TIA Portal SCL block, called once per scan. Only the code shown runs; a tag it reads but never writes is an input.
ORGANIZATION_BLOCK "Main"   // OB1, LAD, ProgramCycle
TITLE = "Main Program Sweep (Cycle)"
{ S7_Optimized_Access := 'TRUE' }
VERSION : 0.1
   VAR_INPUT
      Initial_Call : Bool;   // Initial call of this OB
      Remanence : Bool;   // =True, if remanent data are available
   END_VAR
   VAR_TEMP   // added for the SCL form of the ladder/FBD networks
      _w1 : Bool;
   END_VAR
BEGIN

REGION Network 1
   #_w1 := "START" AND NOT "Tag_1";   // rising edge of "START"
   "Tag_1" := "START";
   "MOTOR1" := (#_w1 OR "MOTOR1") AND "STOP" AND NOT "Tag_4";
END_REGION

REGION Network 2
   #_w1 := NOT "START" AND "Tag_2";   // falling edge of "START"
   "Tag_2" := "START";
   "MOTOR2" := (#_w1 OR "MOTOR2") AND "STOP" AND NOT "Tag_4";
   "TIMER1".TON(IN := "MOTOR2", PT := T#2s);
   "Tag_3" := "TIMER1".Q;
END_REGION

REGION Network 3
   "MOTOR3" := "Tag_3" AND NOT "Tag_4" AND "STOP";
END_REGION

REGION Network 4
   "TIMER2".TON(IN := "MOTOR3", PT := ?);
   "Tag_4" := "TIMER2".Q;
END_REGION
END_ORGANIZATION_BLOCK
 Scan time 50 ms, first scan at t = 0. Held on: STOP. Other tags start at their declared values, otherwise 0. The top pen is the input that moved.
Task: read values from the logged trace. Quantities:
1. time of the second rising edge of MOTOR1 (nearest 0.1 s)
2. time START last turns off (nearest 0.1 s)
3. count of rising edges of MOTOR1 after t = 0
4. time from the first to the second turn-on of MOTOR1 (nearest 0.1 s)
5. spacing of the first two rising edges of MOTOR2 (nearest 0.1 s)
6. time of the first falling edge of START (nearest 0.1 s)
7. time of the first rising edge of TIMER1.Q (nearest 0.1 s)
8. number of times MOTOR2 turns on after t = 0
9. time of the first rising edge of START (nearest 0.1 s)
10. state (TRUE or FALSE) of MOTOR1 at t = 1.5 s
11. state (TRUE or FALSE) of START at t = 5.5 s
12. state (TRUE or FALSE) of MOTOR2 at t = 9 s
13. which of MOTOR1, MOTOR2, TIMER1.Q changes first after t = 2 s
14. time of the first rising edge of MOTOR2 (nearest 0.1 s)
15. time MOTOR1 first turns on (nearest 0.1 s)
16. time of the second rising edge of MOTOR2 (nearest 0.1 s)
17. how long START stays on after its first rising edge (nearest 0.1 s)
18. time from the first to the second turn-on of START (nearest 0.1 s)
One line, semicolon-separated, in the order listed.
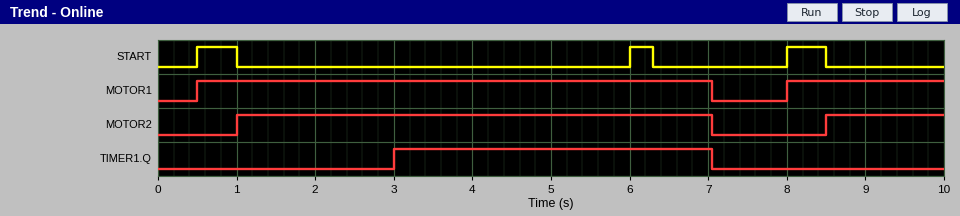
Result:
8.0 s; 8.5 s; 2; 7.5 s; 7.5 s; 1.0 s; 3.0 s; 2; 0.5 s; TRUE; FALSE; TRUE; TIMER1.Q; 1.0 s; 0.5 s; 8.5 s; 0.5 s; 5.5 s
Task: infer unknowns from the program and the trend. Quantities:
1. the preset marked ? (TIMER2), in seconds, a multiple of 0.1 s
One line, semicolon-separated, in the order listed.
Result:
4.0 s
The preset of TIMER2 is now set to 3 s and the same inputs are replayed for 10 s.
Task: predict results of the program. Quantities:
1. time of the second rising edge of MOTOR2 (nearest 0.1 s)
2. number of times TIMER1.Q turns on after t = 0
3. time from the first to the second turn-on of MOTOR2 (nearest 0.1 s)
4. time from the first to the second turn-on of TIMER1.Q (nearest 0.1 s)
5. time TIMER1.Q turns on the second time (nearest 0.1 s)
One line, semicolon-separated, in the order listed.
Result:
6.3 s; 2; 5.3 s; 5.3 s; 8.3 s
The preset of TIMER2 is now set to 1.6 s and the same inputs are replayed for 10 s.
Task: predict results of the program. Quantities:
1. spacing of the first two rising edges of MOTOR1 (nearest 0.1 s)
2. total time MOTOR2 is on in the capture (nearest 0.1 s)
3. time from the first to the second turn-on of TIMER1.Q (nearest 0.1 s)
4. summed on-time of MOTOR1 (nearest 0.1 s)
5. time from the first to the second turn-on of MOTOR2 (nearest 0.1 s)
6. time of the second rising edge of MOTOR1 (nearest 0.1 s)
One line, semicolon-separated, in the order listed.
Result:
5.5 s; 7.3 s; 5.3 s; 8.1 s; 5.3 s; 6.0 s
